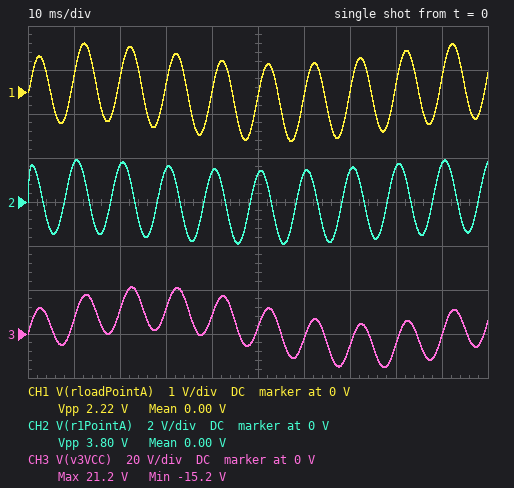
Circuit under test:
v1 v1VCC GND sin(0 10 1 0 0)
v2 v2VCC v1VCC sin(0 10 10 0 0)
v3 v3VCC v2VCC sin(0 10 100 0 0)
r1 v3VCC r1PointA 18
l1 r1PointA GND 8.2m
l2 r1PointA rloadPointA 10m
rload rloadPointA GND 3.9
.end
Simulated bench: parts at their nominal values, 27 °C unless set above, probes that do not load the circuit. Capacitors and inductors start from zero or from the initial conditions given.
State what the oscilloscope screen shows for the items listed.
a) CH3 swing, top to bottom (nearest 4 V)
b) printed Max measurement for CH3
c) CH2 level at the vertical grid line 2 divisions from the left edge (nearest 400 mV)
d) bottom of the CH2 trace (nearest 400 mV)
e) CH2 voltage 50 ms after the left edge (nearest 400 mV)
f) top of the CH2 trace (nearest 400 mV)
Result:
36 V
21.2 V
1.6 V
-2.0 V
1.2 V
2.0 V
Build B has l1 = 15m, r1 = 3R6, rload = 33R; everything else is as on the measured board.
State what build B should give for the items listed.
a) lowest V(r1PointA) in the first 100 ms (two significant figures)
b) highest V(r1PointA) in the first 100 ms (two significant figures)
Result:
-11 V
11 V
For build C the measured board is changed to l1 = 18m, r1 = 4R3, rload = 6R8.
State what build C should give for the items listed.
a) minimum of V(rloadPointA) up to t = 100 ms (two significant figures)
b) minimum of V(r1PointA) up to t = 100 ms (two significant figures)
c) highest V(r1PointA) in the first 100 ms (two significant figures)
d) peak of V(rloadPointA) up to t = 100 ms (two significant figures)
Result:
-7.0 V
-8.8 V
8.5 V
6.7 V
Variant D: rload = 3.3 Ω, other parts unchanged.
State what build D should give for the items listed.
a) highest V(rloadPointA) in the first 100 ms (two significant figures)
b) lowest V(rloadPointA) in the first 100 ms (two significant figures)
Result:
970 mV
-1.0 V
